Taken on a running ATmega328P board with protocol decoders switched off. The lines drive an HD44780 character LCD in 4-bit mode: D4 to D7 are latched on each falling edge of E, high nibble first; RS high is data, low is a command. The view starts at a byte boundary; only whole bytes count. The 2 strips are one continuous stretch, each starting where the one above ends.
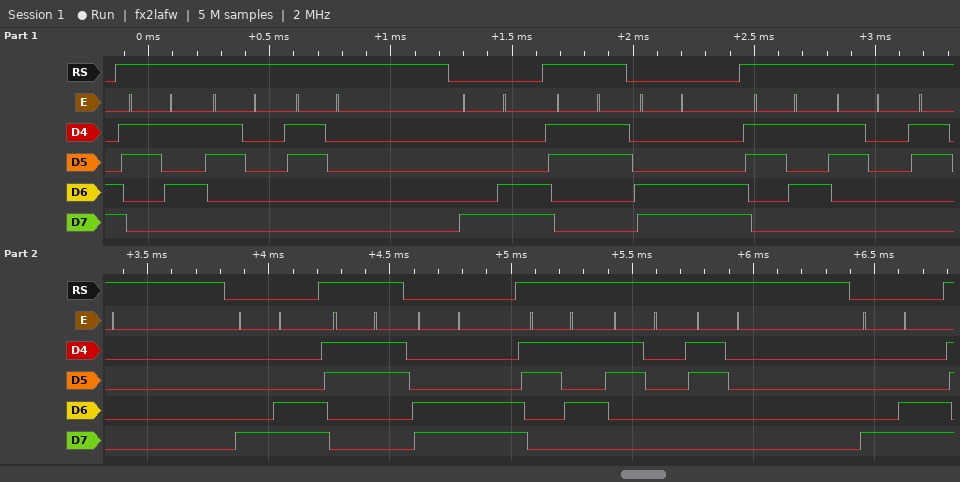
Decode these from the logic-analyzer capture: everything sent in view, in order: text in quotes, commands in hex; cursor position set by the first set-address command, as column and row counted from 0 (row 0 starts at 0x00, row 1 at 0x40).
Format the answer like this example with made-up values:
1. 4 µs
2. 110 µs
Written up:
1. "500" 0x8C "3" 0xCC "500" 0x8C "3" 0xCC "500" 0x8C
2. column 12, row 0
